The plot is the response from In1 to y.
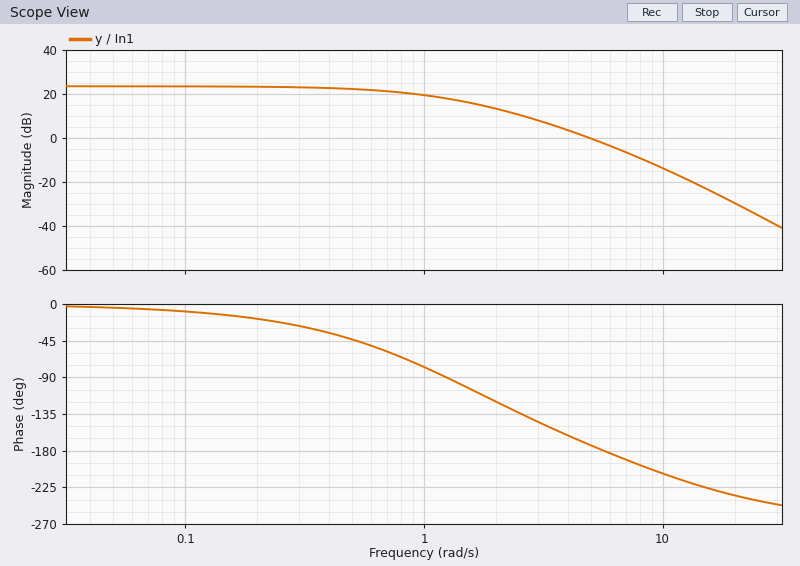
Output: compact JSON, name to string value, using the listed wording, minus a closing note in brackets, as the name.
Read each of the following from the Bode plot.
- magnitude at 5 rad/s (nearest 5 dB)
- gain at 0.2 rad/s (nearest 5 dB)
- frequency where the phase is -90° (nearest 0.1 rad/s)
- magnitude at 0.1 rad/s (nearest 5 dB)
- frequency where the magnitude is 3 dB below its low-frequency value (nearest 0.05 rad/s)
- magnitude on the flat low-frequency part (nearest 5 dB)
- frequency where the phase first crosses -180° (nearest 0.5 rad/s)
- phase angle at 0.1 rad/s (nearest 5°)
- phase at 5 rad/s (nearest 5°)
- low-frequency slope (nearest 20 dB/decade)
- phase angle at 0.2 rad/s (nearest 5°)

{"magnitude at 5 rad/s": "0 dB", "gain at 0.2 rad/s": "25 dB", "frequency where the phase is -90°": "1.2 rad/s", "magnitude at 0.1 rad/s": "25 dB", "frequency where the magnitude is 3 dB below its low-frequency value": "0.85 rad/s", "magnitude on the flat low-frequency part": "25 dB", "frequency where the phase first crosses -180°": "5.5 rad/s", "phase angle at 0.1 rad/s": "-10°", "phase at 5 rad/s": "-175°", "low-frequency slope": "0 dB/decade", "phase angle at 0.2 rad/s": "-20°"}
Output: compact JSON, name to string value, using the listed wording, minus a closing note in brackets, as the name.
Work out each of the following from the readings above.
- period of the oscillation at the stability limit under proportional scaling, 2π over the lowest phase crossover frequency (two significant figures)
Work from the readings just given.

{"period of the oscillation at the stability limit under proportional scaling, 2π over the lowest phase crossover frequency": "1.1 s"}
